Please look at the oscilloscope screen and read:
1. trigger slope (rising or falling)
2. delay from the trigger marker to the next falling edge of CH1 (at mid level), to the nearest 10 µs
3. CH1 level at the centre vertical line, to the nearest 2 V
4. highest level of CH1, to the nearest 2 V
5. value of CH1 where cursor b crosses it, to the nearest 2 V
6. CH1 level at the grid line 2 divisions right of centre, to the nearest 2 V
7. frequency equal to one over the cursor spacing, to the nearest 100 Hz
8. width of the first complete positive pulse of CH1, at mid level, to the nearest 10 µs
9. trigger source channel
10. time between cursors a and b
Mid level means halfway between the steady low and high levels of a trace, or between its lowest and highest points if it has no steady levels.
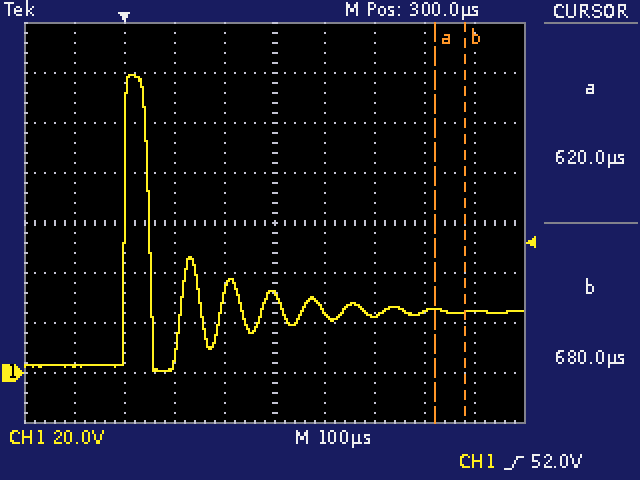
rising
50 µs
32 V
120 V
24 V
22 V
16.7 kHz
50 µs
CH1
60 µs
